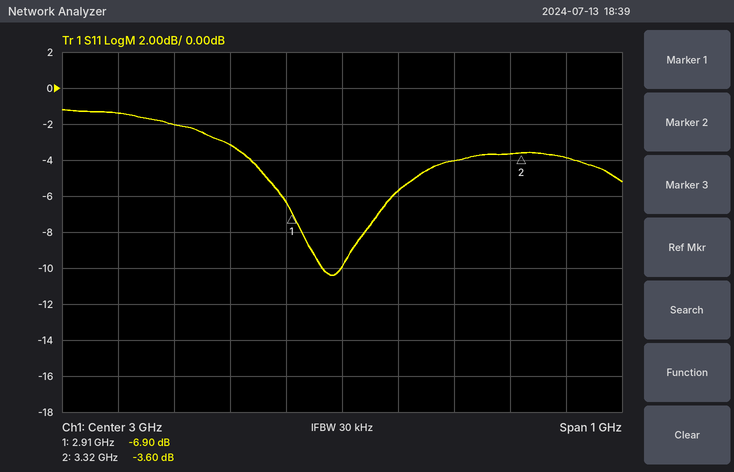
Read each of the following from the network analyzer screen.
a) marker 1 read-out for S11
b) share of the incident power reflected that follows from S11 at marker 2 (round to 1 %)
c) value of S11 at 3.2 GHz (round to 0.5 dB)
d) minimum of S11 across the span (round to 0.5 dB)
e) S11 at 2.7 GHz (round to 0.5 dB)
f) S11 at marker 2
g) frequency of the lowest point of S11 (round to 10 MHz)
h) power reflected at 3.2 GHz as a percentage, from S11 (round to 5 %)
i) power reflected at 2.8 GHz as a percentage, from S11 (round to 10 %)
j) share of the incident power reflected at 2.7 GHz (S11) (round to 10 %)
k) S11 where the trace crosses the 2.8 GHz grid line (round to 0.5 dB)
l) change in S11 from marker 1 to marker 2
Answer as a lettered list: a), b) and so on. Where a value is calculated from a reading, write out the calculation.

a) -6.90 dB
b) 10^(-3.6/10) ≈ 44 %
c) -4.0 dB
d) -10.5 dB
e) -2.0 dB
f) -3.60 dB
g) 2.98 GHz
h) 10^(-4/10) ≈ 40 %
i) 10^(-3/10) ≈ 50 %
j) 10^(-2/10) ≈ 63.1 %, so 60 % to the nearest 10 %
k) -3.0 dB
l) -3.6 − (-6.9) = 3.30 dB
